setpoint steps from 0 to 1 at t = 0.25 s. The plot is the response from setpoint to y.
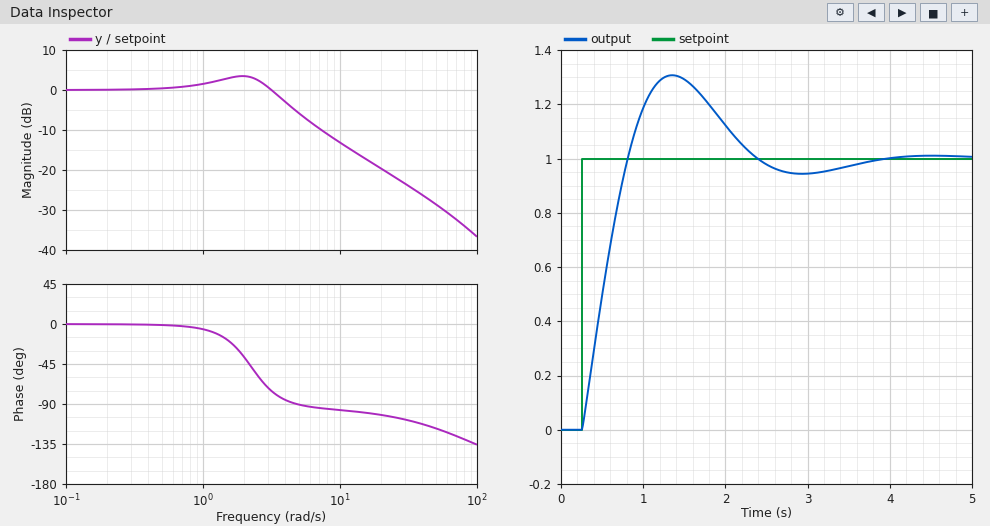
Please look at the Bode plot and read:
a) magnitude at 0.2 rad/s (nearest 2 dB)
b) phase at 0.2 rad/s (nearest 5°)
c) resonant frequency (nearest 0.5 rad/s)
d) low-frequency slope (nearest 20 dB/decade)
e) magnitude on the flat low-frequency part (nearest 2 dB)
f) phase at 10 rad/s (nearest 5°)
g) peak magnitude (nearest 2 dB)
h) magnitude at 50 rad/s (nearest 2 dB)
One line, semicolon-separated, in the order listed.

0 dB; 0°; 2.0 rad/s; 0 dB/decade; 0 dB; -95°; 4 dB; -28 dB
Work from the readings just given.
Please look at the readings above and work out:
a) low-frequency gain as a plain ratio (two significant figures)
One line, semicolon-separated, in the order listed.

1.0
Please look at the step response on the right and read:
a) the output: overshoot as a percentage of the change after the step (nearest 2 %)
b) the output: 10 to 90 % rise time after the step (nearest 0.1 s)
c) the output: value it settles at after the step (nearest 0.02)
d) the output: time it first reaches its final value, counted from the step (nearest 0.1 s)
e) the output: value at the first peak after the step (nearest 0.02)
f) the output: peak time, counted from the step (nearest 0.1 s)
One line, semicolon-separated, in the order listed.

30 %; 0.4 s; 1.00; 0.6 s; 1.30; 1.1 s
